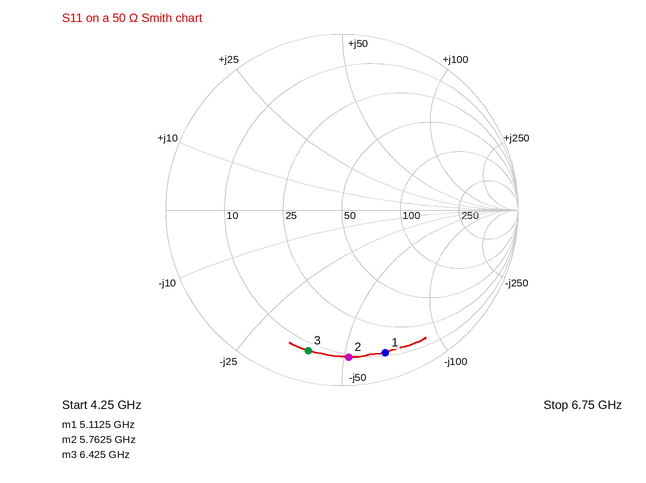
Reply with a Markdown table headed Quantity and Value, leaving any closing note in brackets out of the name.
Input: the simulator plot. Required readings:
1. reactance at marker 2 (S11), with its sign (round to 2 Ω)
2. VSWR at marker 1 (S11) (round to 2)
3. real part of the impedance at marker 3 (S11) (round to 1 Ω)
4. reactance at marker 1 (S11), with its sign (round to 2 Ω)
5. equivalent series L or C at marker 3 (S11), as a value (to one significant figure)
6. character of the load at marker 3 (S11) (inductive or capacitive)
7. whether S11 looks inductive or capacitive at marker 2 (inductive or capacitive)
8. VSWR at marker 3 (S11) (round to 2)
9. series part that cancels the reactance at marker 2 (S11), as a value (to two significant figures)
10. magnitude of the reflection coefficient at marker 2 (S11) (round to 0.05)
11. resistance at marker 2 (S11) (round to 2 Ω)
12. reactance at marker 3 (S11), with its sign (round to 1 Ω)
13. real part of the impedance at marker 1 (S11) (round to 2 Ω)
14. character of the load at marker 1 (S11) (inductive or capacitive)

| Quantity | Value |
|---|---|
| reactance at marker 2 (S11), with its sign | -52 Ω |
| VSWR at marker 1 (S11) | 12 |
| real part of the impedance at marker 3 (S11) | 8 Ω |
| reactance at marker 1 (S11), with its sign | -66 Ω |
| equivalent series L or C at marker 3 (S11), as a value | 600 fF |
| character of the load at marker 3 (S11) | capacitive |
| whether S11 looks inductive or capacitive at marker 2 | capacitive |
| VSWR at marker 3 (S11) | 10 |
| series part that cancels the reactance at marker 2 (S11), as a value | 1.4 nH |
| magnitude of the reflection coefficient at marker 2 (S11) | 0.85 |
| resistance at marker 2 (S11) | 10 Ω |
| reactance at marker 3 (S11), with its sign | -39 Ω |
| real part of the impedance at marker 1 (S11) | 12 Ω |
| character of the load at marker 1 (S11) | capacitive |
